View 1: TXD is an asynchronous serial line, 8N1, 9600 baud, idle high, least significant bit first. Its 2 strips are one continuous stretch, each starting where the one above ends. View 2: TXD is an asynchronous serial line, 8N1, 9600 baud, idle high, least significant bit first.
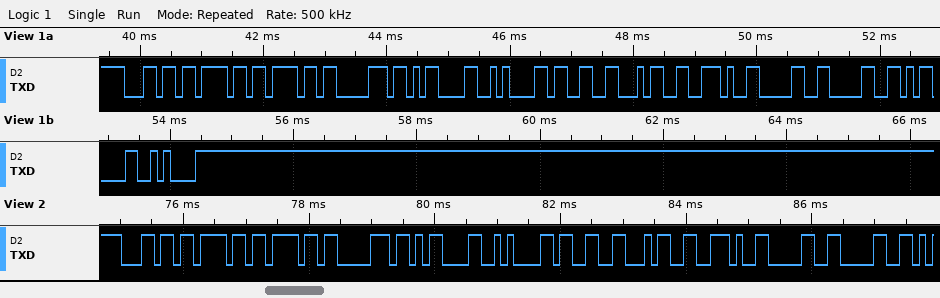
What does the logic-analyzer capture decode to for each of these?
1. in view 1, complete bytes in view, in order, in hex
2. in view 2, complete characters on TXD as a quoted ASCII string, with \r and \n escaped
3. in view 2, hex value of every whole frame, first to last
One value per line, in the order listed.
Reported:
6C 6F 6F 70 0D 0A 33 34 2E 30 30 0D 0A
"loop\r\n34.00"
6C 6F 6F 70 0D 0A 33 34 2E 30 30
